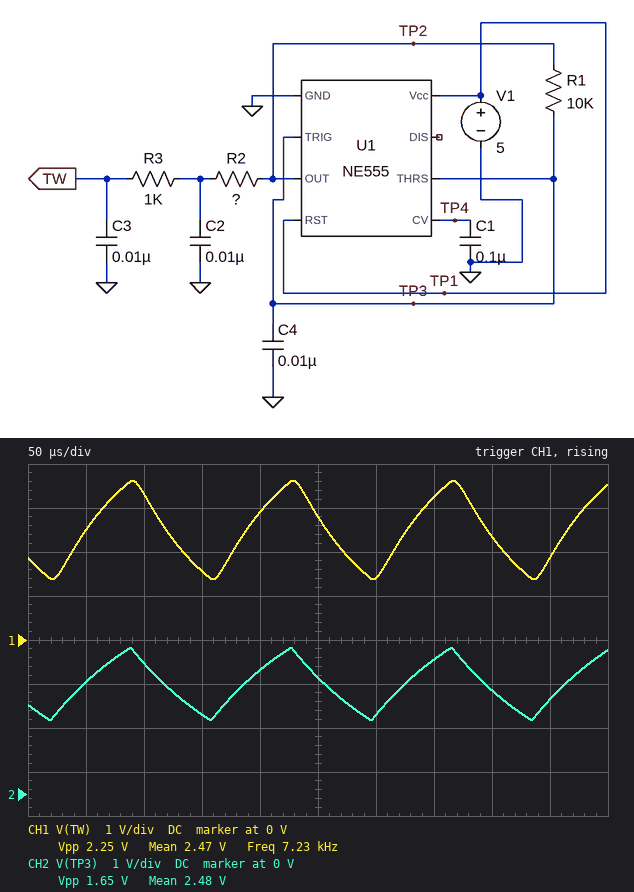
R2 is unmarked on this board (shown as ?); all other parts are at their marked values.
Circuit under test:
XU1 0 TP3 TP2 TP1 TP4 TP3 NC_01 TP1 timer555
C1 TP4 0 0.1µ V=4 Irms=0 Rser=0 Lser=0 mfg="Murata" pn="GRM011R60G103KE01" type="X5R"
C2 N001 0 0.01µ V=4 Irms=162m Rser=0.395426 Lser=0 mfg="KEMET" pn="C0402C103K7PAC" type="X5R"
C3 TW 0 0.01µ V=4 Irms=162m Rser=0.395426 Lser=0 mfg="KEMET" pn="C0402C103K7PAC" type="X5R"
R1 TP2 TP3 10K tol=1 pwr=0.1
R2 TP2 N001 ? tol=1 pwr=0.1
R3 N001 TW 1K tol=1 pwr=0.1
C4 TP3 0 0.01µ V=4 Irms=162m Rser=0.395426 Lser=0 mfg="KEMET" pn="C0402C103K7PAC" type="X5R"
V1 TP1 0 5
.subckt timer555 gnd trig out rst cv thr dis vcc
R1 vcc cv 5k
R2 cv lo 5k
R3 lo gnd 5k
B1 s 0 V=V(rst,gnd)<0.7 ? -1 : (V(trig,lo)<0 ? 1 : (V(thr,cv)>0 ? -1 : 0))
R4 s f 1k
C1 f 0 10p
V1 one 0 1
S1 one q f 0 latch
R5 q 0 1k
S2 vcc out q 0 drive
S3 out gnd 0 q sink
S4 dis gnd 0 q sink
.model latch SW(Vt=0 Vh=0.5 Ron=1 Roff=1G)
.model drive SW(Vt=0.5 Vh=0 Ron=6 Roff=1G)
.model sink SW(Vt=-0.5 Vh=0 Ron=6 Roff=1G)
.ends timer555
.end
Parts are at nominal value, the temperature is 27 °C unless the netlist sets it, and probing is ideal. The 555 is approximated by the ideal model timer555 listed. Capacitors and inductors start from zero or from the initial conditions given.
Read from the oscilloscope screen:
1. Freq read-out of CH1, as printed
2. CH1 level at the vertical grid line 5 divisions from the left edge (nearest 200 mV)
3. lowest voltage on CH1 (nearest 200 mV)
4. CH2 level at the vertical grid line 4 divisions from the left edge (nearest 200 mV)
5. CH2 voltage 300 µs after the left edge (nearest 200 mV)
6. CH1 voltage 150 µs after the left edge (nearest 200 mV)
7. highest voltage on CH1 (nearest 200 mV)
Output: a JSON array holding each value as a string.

["7.23 kHz", "2.8 V", "1.4 V", "2.8 V", "1.8 V", "1.6 V", "3.6 V"]
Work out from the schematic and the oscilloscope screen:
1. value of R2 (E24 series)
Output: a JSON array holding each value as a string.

["3 kΩ"]
